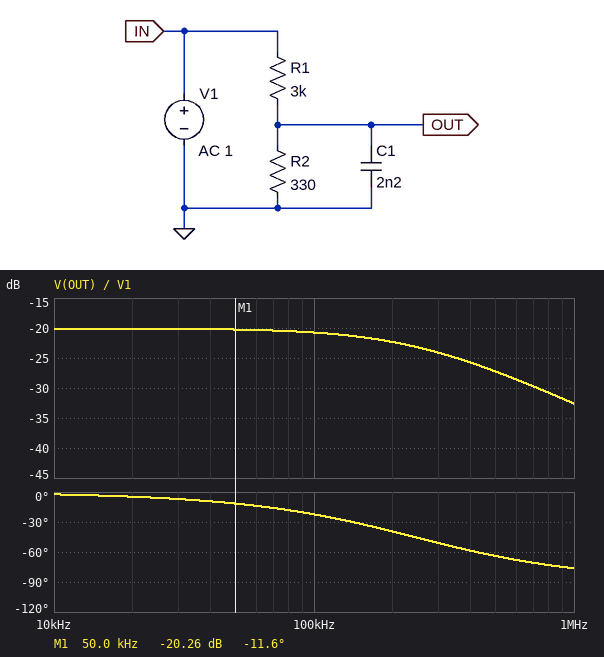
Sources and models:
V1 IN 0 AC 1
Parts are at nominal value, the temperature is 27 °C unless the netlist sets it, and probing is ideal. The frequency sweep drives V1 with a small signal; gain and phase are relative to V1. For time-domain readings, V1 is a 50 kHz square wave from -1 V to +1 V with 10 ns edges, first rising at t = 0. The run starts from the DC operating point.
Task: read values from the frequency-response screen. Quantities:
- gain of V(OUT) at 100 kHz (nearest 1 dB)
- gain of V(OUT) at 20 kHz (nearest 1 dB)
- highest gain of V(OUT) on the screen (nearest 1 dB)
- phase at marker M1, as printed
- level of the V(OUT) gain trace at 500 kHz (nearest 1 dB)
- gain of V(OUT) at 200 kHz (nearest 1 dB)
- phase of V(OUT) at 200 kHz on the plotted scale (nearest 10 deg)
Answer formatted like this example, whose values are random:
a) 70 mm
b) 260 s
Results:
a) -21 dB
b) -20 dB
c) -20 dB
d) -11.6 deg
e) -27 dB
f) -22 dB
g) -40 deg
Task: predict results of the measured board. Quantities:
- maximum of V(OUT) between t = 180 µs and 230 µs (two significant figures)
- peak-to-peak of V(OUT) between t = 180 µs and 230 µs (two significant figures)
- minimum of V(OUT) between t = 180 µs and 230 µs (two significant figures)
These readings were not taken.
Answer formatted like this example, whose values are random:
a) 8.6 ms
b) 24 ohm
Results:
a) 99 mV
b) 200 mV
c) -99 mV
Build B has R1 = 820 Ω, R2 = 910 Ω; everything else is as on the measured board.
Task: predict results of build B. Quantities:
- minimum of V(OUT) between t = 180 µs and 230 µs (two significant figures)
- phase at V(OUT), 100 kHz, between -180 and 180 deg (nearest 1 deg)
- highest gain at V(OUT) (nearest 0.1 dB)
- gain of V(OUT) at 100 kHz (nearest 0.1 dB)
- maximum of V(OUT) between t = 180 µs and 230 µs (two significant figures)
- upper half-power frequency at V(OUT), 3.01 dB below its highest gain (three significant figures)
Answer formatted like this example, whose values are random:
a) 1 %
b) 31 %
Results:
a) -530 mV
b) -31 deg
c) -5.6 dB
d) -6.9 dB
e) 530 mV
f) 168 kHz
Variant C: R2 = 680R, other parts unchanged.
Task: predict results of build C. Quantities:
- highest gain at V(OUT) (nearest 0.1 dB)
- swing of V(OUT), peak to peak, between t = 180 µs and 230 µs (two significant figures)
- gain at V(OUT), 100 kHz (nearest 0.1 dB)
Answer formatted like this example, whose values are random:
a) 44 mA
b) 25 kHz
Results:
a) -14.7 dB
b) 370 mV
c) -16.7 dB
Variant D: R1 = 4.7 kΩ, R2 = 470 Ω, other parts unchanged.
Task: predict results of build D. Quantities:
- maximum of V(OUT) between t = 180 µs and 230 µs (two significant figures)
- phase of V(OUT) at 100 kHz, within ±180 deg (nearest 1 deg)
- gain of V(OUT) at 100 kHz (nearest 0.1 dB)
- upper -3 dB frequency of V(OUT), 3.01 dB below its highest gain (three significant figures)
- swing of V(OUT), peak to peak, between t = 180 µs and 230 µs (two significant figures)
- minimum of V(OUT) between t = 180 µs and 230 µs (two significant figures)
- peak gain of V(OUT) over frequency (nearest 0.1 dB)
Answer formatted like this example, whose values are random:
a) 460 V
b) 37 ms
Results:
a) 91 mV
b) -31 deg
c) -22.1 dB
d) 169 kHz
e) 180 mV
f) -91 mV
g) -20.8 dB
